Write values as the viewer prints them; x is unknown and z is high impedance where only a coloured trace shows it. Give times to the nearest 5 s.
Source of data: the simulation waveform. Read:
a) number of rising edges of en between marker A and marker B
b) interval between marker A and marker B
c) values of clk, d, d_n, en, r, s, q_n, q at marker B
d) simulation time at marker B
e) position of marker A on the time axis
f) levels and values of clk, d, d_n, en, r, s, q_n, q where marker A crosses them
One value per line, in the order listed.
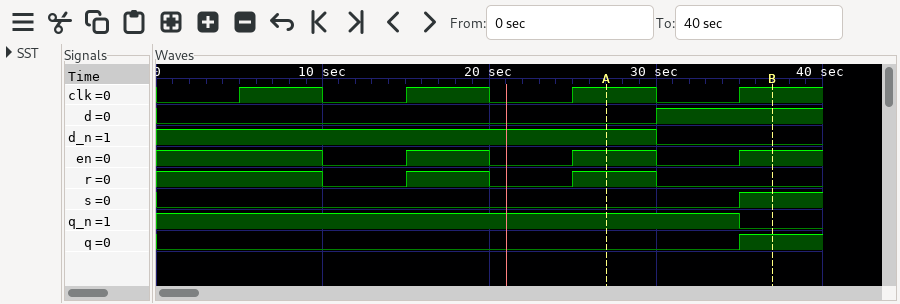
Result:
1
10 s
clk=1, d=1, d_n=0, en=1, r=0, s=1, q_n=0, q=1
35 s
25 s
clk=1, d=0, d_n=1, en=1, r=1, s=0, q_n=1, q=0
